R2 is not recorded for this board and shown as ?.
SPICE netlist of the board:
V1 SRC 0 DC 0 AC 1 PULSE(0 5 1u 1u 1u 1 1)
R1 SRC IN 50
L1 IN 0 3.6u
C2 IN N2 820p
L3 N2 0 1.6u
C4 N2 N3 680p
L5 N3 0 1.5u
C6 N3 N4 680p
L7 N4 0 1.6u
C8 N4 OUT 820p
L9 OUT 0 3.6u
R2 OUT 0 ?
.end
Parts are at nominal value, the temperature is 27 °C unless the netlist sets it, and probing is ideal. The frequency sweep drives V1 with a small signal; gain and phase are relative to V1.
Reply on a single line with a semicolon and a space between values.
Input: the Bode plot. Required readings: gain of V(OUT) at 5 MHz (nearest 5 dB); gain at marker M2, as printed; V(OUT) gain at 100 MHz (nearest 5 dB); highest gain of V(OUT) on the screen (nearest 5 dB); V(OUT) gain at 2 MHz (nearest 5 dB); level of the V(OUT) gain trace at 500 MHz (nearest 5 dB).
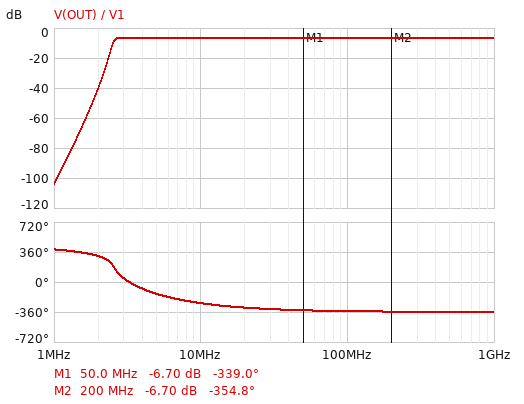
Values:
-5 dB; -6.70 dB; -5 dB; -5 dB; -40 dB; -5 dB
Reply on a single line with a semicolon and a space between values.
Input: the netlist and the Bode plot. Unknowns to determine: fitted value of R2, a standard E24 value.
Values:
43 Ω
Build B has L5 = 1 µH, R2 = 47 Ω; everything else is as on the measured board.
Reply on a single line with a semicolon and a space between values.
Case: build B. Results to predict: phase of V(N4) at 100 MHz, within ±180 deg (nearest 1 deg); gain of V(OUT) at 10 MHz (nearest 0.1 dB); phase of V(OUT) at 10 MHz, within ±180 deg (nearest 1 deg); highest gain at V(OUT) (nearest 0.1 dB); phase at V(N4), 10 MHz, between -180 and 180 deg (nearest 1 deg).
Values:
9 deg; -6.4 dB; 113 deg; -6.3 dB; 89 deg
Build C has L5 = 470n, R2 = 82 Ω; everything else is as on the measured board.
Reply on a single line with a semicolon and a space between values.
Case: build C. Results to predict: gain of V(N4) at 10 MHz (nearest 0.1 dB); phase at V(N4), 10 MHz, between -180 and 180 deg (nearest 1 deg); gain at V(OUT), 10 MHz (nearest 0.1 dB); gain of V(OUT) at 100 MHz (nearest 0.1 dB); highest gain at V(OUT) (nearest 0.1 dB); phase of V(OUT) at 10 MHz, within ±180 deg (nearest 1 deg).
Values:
-6.7 dB; 115 deg; -6.2 dB; -4.2 dB; -4.1 dB; 130 deg
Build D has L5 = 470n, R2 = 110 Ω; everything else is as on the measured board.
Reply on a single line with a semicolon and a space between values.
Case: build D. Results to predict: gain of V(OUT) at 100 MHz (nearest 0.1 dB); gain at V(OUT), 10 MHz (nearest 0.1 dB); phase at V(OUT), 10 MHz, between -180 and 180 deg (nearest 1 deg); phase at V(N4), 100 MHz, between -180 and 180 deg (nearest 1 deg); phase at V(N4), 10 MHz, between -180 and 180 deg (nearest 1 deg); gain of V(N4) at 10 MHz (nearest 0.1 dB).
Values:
-3.3 dB; -5.7 dB; 128 deg; 14 deg; 117 deg; -6.3 dB
